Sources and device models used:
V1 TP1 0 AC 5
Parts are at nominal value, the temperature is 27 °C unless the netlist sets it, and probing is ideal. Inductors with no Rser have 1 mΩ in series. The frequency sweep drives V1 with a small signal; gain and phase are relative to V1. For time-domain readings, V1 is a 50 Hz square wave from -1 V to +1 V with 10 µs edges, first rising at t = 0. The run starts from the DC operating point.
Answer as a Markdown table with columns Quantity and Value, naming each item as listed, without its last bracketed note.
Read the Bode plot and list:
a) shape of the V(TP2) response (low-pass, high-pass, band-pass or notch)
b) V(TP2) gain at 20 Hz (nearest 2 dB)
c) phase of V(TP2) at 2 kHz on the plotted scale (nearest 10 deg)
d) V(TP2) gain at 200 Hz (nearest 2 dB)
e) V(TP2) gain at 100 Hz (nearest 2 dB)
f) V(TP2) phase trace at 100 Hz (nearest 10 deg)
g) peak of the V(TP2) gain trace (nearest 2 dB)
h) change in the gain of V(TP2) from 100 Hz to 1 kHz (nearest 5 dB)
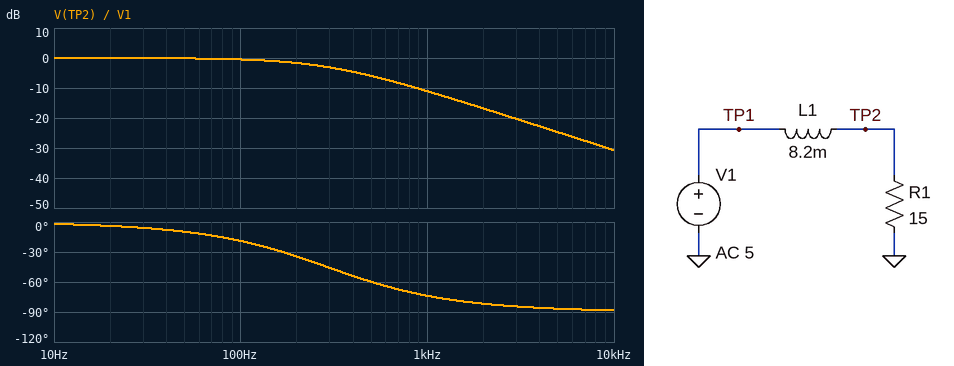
| Quantity | Value |
|---|---|
| shape of the V(TP2) response | low-pass |
| V(TP2) gain at 20 Hz | 0 dB |
| phase of V(TP2) at 2 kHz on the plotted scale | -80 deg |
| V(TP2) gain at 200 Hz | -2 dB |
| V(TP2) gain at 100 Hz | 0 dB |
| V(TP2) phase trace at 100 Hz | -20 deg |
| peak of the V(TP2) gain trace | 0 dB |
| change in the gain of V(TP2) from 100 Hz to 1 kHz | -10 dB |
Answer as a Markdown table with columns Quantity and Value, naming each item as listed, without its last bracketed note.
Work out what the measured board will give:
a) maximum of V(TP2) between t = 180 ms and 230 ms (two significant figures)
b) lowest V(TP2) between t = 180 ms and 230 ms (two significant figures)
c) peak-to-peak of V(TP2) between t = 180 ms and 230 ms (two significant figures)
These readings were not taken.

| Quantity | Value |
|---|---|
| maximum of V(TP2) between t = 180 ms and 230 ms | 1.0 V |
| lowest V(TP2) between t = 180 ms and 230 ms | -1.0 V |
| peak-to-peak of V(TP2) between t = 180 ms and 230 ms | 2.0 V |
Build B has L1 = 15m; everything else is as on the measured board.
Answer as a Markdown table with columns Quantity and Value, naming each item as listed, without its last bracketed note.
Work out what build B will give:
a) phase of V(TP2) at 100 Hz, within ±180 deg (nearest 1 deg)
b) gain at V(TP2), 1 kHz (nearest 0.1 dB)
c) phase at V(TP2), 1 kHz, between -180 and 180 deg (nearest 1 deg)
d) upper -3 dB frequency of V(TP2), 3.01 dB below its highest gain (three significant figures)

| Quantity | Value |
|---|---|
| phase of V(TP2) at 100 Hz, within ±180 deg | -32 deg |
| gain at V(TP2), 1 kHz | -16.1 dB |
| phase at V(TP2), 1 kHz, between -180 and 180 deg | -81 deg |
| upper -3 dB frequency of V(TP2), 3.01 dB below its highest gain | 159 Hz |
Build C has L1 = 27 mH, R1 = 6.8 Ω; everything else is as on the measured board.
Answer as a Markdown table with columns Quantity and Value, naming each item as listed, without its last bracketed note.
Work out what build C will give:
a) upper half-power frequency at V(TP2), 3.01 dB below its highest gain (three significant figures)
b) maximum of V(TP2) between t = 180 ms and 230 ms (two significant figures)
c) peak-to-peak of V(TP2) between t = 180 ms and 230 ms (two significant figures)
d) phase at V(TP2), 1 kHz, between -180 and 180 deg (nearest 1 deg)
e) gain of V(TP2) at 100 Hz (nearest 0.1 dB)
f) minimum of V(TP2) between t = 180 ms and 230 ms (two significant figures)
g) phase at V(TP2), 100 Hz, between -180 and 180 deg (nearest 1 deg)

| Quantity | Value |
|---|---|
| upper half-power frequency at V(TP2), 3.01 dB below its highest gain | 40.1 Hz |
| maximum of V(TP2) between t = 180 ms and 230 ms | 850 mV |
| peak-to-peak of V(TP2) between t = 180 ms and 230 ms | 1.7 V |
| phase at V(TP2), 1 kHz, between -180 and 180 deg | -88 deg |
| gain of V(TP2) at 100 Hz | -8.6 dB |
| minimum of V(TP2) between t = 180 ms and 230 ms | -850 mV |
| phase at V(TP2), 100 Hz, between -180 and 180 deg | -68 deg |
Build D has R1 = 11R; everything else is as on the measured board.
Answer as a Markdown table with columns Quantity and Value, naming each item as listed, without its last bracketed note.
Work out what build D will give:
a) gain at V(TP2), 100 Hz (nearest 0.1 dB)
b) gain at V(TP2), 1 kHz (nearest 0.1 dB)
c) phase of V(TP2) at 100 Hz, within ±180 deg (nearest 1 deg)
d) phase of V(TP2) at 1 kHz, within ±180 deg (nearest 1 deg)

| Quantity | Value |
|---|---|
| gain at V(TP2), 100 Hz | -0.9 dB |
| gain at V(TP2), 1 kHz | -13.6 dB |
| phase of V(TP2) at 100 Hz, within ±180 deg | -25 deg |
| phase of V(TP2) at 1 kHz, within ±180 deg | -78 deg |
